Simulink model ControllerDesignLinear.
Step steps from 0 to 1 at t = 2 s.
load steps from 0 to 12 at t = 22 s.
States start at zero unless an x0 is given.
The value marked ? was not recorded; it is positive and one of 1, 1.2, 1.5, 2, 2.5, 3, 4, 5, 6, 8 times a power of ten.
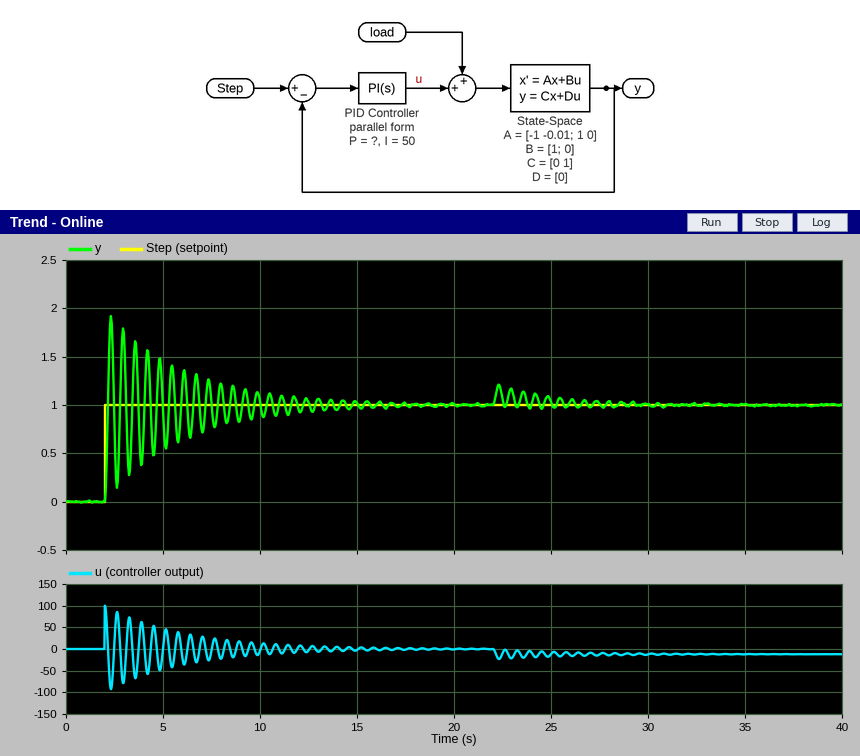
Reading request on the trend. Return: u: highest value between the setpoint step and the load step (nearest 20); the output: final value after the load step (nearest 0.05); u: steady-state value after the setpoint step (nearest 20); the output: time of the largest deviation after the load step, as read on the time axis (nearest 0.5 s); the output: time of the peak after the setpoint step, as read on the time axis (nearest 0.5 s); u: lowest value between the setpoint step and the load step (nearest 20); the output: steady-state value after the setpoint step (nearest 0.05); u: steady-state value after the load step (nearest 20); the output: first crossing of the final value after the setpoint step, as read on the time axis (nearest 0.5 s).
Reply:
100
1.00
0
22.5 s
2.5 s
-100
1.00
-20
2.0 s
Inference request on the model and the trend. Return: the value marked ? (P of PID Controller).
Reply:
100
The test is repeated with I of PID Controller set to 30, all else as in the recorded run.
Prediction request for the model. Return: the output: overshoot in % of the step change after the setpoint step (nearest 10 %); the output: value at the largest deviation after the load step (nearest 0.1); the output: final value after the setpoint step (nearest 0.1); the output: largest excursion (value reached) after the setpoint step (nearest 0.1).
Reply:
90 %
1.2
1.0
1.9
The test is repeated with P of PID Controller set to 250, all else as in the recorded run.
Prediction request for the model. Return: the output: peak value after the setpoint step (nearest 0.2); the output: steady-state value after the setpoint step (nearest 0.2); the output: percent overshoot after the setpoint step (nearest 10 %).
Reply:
2.0
1.0
90 %
